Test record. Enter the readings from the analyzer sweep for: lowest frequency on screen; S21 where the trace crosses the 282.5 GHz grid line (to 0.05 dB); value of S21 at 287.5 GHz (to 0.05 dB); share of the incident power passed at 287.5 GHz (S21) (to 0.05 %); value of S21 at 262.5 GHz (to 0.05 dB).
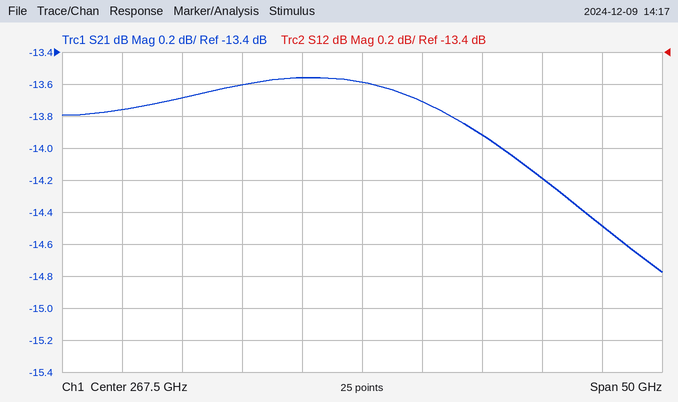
242.5 GHz
-14.20 dB
-14.50 dB
3.55 %
-13.55 dB
